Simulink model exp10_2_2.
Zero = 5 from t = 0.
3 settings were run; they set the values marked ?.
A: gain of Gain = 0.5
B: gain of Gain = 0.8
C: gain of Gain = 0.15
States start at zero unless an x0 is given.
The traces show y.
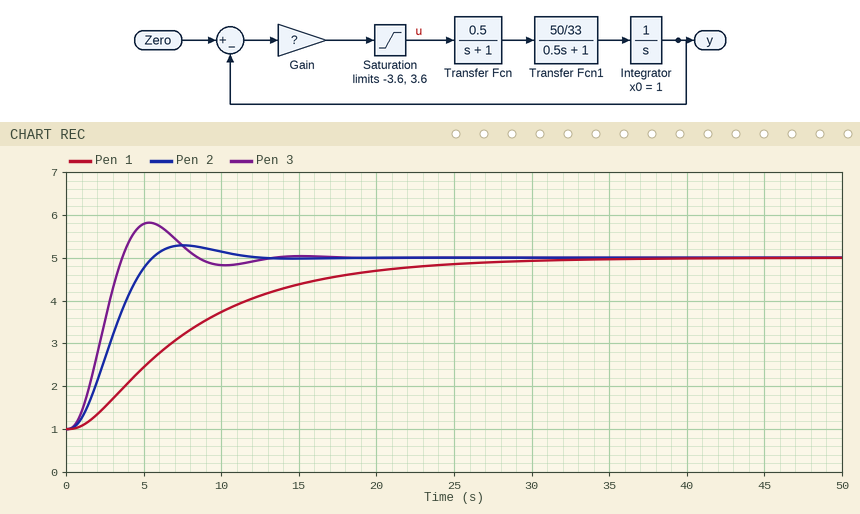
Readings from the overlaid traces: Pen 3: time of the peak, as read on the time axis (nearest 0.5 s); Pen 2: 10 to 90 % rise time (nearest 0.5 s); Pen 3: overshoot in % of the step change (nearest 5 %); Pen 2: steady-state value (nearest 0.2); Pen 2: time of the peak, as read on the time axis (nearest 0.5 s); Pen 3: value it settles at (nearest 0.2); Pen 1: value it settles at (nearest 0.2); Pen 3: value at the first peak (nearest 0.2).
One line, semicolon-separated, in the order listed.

5.5 s; 3.5 s; 20 %; 5.0; 7.5 s; 5.0; 5.0; 5.8
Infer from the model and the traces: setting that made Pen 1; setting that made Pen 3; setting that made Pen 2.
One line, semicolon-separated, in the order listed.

C; B; A
